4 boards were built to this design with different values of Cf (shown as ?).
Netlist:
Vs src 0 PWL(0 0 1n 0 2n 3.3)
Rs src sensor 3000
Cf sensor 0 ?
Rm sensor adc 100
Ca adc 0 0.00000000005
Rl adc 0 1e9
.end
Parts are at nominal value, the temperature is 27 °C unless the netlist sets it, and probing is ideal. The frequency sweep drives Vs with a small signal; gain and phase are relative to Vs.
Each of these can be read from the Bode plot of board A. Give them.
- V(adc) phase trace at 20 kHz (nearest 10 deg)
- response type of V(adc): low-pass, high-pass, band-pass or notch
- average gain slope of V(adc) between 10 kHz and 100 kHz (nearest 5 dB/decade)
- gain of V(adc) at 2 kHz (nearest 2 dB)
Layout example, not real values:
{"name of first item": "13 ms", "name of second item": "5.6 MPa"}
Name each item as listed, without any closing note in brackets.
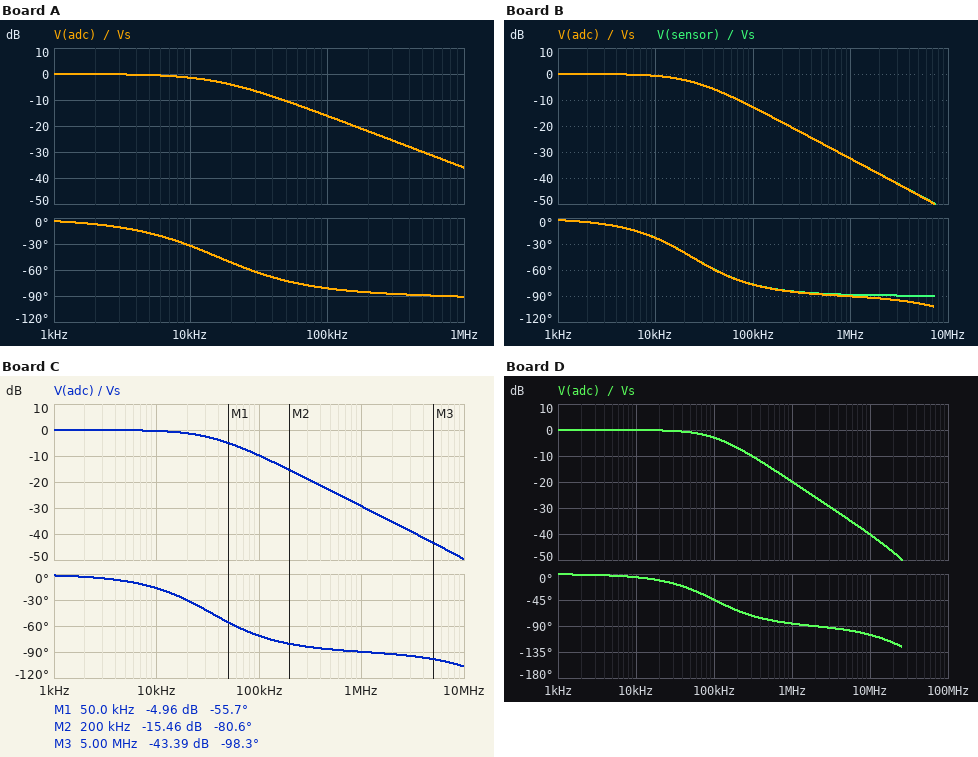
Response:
{"V(adc) phase trace at 20 kHz": "-50 deg", "response type of V(adc): low-pass, high-pass, band-pass or notch": "low-pass", "average gain slope of V(adc) between 10 kHz and 100 kHz": "-15 dB/decade", "gain of V(adc) at 2 kHz": "0 dB"}
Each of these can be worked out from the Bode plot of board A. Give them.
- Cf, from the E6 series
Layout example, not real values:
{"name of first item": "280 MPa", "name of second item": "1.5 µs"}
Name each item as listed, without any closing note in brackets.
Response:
{"Cf, from the E6 series": "3.3 nF"}
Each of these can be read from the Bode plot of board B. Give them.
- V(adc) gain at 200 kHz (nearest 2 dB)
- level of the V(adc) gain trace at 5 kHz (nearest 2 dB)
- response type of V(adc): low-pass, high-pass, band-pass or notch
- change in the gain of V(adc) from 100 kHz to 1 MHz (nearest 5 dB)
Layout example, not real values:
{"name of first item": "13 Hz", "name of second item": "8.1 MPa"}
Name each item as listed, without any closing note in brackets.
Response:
{"V(adc) gain at 200 kHz": "-18 dB", "level of the V(adc) gain trace at 5 kHz": "0 dB", "response type of V(adc): low-pass, high-pass, band-pass or notch": "low-pass", "change in the gain of V(adc) from 100 kHz to 1 MHz": "-20 dB"}
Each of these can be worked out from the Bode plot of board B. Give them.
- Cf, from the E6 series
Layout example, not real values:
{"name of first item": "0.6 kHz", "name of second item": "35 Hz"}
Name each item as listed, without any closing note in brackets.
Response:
{"Cf, from the E6 series": "2.2 nF"}
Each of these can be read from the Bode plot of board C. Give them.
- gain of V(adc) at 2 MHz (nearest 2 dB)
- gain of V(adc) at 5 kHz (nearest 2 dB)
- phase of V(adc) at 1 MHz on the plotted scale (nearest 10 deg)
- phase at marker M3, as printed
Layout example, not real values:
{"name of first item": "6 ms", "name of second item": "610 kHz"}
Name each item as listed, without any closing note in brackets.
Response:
{"gain of V(adc) at 2 MHz": "-36 dB", "gain of V(adc) at 5 kHz": "0 dB", "phase of V(adc) at 1 MHz on the plotted scale": "-90 deg", "phase at marker M3, as printed": "-98.3 deg"}
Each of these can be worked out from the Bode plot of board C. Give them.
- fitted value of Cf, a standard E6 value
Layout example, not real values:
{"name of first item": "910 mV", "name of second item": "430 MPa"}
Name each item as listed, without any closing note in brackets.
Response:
{"fitted value of Cf, a standard E6 value": "1.5 nF"}
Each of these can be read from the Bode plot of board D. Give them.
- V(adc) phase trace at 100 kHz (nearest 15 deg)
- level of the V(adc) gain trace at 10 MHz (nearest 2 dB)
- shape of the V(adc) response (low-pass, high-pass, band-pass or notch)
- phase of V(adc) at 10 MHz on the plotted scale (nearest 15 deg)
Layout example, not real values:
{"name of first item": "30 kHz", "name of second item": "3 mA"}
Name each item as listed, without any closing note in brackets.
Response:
{"V(adc) phase trace at 100 kHz": "-45 deg", "level of the V(adc) gain trace at 10 MHz": "-40 dB", "shape of the V(adc) response": "low-pass", "phase of V(adc) at 10 MHz on the plotted scale": "-105 deg"}
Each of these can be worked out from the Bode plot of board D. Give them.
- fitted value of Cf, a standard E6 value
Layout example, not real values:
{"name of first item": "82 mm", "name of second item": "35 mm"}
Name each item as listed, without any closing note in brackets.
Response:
{"fitted value of Cf, a standard E6 value": "470 pF"}
